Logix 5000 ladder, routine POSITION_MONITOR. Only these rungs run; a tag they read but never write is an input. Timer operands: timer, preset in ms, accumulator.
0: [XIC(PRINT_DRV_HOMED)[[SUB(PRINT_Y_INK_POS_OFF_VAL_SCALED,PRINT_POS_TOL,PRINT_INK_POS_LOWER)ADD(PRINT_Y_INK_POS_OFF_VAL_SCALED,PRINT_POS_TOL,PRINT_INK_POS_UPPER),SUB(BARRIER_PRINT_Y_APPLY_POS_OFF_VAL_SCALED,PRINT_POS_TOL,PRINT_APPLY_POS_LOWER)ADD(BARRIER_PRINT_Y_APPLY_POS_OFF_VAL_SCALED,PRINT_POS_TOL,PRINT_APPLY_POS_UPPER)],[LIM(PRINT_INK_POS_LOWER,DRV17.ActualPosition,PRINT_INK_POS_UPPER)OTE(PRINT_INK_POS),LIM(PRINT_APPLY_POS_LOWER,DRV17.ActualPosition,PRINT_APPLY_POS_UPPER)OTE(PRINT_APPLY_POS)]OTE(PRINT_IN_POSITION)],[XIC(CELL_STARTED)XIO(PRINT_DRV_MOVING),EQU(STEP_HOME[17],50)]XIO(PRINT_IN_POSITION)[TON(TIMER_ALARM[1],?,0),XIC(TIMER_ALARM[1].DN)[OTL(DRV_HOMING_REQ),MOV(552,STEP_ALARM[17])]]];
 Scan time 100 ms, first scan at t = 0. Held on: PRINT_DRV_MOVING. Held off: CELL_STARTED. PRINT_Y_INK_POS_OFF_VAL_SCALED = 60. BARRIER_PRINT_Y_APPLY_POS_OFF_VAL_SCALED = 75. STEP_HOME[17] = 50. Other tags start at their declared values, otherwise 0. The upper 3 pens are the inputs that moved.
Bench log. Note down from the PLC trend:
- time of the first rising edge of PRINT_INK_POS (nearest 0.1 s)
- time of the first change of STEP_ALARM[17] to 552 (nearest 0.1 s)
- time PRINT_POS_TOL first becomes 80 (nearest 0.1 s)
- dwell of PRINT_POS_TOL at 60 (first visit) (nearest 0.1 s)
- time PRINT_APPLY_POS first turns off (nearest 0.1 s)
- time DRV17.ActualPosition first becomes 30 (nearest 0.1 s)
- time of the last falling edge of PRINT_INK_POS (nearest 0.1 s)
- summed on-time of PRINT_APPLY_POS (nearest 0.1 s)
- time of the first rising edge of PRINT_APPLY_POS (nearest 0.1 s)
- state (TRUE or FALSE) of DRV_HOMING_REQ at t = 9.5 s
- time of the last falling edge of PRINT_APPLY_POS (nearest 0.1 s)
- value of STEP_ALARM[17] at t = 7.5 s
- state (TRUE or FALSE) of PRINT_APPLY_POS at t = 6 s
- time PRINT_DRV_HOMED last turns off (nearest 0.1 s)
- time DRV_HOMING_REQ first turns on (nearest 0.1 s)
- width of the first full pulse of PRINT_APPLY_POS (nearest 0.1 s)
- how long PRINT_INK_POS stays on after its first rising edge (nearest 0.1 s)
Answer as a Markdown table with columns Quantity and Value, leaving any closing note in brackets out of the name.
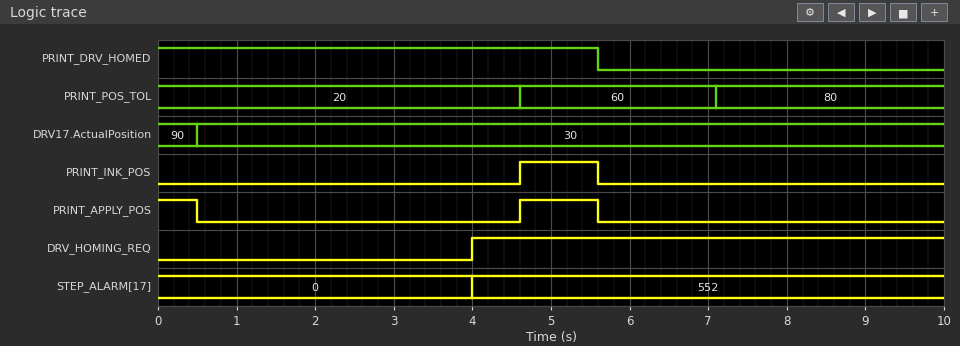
| Quantity | Value |
|---|---|
| time of the first rising edge of PRINT_INK_POS | 4.6 s |
| time of the first change of STEP_ALARM[17] to 552 | 4.0 s |
| time PRINT_POS_TOL first becomes 80 | 7.1 s |
| dwell of PRINT_POS_TOL at 60 (first visit) | 2.5 s |
| time PRINT_APPLY_POS first turns off | 0.5 s |
| time DRV17.ActualPosition first becomes 30 | 0.5 s |
| time of the last falling edge of PRINT_INK_POS | 5.6 s |
| summed on-time of PRINT_APPLY_POS | 1.5 s |
| time of the first rising edge of PRINT_APPLY_POS | 4.6 s |
| state (TRUE or FALSE) of DRV_HOMING_REQ at t = 9.5 s | TRUE |
| time of the last falling edge of PRINT_APPLY_POS | 5.6 s |
| value of STEP_ALARM[17] at t = 7.5 s | 552 |
| state (TRUE or FALSE) of PRINT_APPLY_POS at t = 6 s | FALSE |
| time PRINT_DRV_HOMED last turns off | 5.6 s |
| time DRV_HOMING_REQ first turns on | 4.0 s |
| width of the first full pulse of PRINT_APPLY_POS | 1.0 s |
| how long PRINT_INK_POS stays on after its first rising edge | 1.0 s |
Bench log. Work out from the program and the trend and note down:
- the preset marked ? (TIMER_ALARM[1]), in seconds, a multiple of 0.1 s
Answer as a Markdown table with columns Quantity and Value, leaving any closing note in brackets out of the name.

| Quantity | Value |
|---|---|
| the preset marked ? (TIMER_ALARM[1]), in seconds, a multiple of 0.1 s | 3.5 s |
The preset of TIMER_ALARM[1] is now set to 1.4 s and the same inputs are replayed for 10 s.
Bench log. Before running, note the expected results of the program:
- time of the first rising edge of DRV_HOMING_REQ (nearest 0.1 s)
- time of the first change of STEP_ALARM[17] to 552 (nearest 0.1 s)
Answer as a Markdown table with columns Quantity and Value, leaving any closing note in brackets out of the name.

| Quantity | Value |
|---|---|
| time of the first rising edge of DRV_HOMING_REQ | 1.9 s |
| time of the first change of STEP_ALARM[17] to 552 | 1.9 s |
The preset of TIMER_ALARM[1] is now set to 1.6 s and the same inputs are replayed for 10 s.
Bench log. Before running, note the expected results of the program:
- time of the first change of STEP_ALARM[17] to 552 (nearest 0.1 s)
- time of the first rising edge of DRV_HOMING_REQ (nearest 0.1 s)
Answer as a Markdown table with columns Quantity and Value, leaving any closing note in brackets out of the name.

| Quantity | Value |
|---|---|
| time of the first change of STEP_ALARM[17] to 552 | 2.1 s |
| time of the first rising edge of DRV_HOMING_REQ | 2.1 s |
